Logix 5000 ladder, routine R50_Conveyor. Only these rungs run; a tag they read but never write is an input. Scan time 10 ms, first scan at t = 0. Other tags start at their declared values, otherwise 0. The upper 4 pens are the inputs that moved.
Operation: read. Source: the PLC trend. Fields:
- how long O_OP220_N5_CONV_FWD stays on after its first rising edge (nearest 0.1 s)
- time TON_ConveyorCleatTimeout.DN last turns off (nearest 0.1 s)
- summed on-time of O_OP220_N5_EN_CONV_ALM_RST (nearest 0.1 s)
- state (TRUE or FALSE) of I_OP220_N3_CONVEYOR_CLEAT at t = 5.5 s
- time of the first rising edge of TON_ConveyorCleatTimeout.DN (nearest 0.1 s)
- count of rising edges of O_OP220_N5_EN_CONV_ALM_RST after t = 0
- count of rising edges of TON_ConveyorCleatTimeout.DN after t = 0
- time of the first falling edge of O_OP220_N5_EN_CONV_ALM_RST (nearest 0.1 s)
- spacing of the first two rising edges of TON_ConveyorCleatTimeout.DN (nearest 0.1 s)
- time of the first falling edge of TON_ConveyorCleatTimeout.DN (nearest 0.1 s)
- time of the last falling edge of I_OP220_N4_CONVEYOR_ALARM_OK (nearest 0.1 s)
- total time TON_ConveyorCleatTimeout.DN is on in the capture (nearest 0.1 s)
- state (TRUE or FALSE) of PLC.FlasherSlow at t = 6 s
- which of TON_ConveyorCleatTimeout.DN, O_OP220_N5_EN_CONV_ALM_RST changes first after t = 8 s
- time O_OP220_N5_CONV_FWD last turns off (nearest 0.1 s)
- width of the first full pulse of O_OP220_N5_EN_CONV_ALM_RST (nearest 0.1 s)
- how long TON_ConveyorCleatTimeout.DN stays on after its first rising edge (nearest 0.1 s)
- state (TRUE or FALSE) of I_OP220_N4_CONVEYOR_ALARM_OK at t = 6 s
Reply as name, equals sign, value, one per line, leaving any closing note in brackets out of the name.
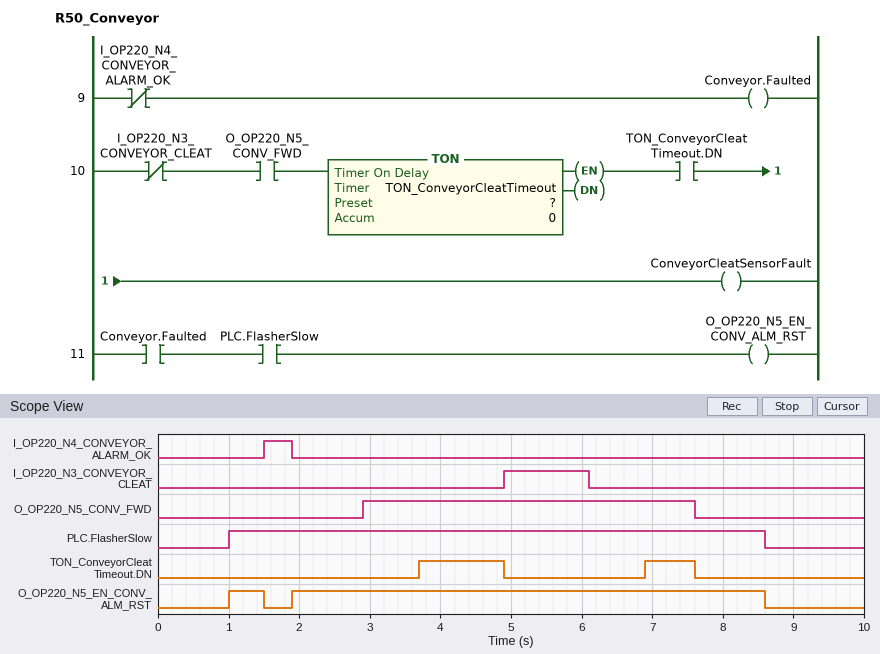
how long O_OP220_N5_CONV_FWD stays on after its first rising edge = 4.7 s
time TON_ConveyorCleatTimeout.DN last turns off = 7.6 s
summed on-time of O_OP220_N5_EN_CONV_ALM_RST = 7.2 s
state (TRUE or FALSE) of I_OP220_N3_CONVEYOR_CLEAT at t = 5.5 s = TRUE
time of the first rising edge of TON_ConveyorCleatTimeout.DN = 3.7 s
count of rising edges of O_OP220_N5_EN_CONV_ALM_RST after t = 0 = 2
count of rising edges of TON_ConveyorCleatTimeout.DN after t = 0 = 2
time of the first falling edge of O_OP220_N5_EN_CONV_ALM_RST = 1.5 s
spacing of the first two rising edges of TON_ConveyorCleatTimeout.DN = 3.2 s
time of the first falling edge of TON_ConveyorCleatTimeout.DN = 4.9 s
time of the last falling edge of I_OP220_N4_CONVEYOR_ALARM_OK = 1.9 s
total time TON_ConveyorCleatTimeout.DN is on in the capture = 1.9 s
state (TRUE or FALSE) of PLC.FlasherSlow at t = 6 s = TRUE
which of TON_ConveyorCleatTimeout.DN, O_OP220_N5_EN_CONV_ALM_RST changes first after t = 8 s = O_OP220_N5_EN_CONV_ALM_RST
time O_OP220_N5_CONV_FWD last turns off = 7.6 s
width of the first full pulse of O_OP220_N5_EN_CONV_ALM_RST = 0.5 s
how long TON_ConveyorCleatTimeout.DN stays on after its first rising edge = 1.2 s
state (TRUE or FALSE) of I_OP220_N4_CONVEYOR_ALARM_OK at t = 6 s = FALSE
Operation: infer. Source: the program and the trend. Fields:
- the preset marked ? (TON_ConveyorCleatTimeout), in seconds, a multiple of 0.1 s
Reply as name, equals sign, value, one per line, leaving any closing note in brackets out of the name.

the preset marked ? (TON_ConveyorCleatTimeout), in seconds, a multiple of 0.1 s = 0.8 s
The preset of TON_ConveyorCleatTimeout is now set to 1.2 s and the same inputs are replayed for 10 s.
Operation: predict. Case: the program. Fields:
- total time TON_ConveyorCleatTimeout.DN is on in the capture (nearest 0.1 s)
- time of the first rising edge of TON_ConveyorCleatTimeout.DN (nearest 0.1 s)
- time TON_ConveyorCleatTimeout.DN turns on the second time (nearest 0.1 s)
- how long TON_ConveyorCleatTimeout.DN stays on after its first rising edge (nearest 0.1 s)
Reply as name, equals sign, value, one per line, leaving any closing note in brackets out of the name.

total time TON_ConveyorCleatTimeout.DN is on in the capture = 1.1 s
time of the first rising edge of TON_ConveyorCleatTimeout.DN = 4.1 s
time TON_ConveyorCleatTimeout.DN turns on the second time = 7.3 s
how long TON_ConveyorCleatTimeout.DN stays on after its first rising edge = 0.8 s
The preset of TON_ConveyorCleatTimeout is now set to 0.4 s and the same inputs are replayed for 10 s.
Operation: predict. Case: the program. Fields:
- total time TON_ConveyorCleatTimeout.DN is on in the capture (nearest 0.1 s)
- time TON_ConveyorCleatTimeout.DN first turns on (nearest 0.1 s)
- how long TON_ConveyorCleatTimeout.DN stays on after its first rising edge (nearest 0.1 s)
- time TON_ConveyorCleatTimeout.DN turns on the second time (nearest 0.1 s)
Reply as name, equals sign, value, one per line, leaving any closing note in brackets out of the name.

total time TON_ConveyorCleatTimeout.DN is on in the capture = 2.7 s
time TON_ConveyorCleatTimeout.DN first turns on = 3.3 s
how long TON_ConveyorCleatTimeout.DN stays on after its first rising edge = 1.6 s
time TON_ConveyorCleatTimeout.DN turns on the second time = 6.5 s
